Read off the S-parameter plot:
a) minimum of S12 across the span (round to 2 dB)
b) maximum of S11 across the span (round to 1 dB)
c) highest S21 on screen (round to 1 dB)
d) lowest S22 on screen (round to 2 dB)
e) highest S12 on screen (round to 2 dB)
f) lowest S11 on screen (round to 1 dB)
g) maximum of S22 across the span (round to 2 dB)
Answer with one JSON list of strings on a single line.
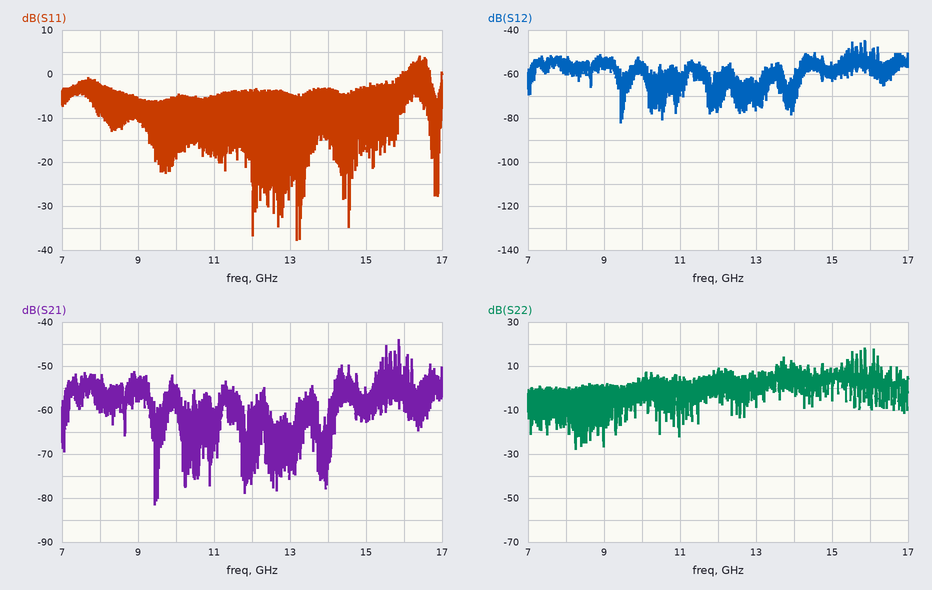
["-82 dB", "4 dB", "-44 dB", "-28 dB", "-44 dB", "-38 dB", "18 dB"]
